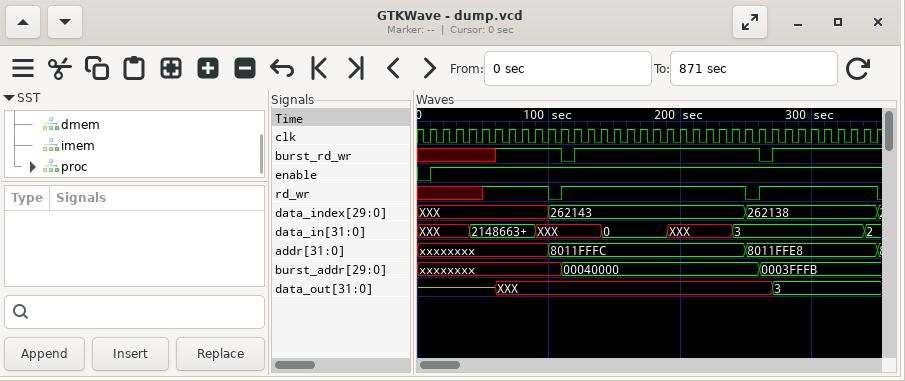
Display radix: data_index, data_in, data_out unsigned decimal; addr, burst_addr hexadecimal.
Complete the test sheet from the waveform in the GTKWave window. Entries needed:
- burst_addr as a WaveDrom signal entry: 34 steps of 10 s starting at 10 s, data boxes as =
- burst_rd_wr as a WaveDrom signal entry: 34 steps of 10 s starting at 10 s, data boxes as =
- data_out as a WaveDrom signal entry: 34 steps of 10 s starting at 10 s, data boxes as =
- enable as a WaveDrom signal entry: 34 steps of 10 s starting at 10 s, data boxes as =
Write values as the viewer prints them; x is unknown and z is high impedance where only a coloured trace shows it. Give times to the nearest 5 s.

{name: 'burst_addr', wave: 'x.........=..............=........', data: '00040000 0003FFFB'}
{name: 'burst_rd_wr', wave: 'x....1....01.............01.......'}
{name: 'data_out', wave: 'z....x....................=.......', data: '3'}
{name: 'enable', wave: '1.................................'}
